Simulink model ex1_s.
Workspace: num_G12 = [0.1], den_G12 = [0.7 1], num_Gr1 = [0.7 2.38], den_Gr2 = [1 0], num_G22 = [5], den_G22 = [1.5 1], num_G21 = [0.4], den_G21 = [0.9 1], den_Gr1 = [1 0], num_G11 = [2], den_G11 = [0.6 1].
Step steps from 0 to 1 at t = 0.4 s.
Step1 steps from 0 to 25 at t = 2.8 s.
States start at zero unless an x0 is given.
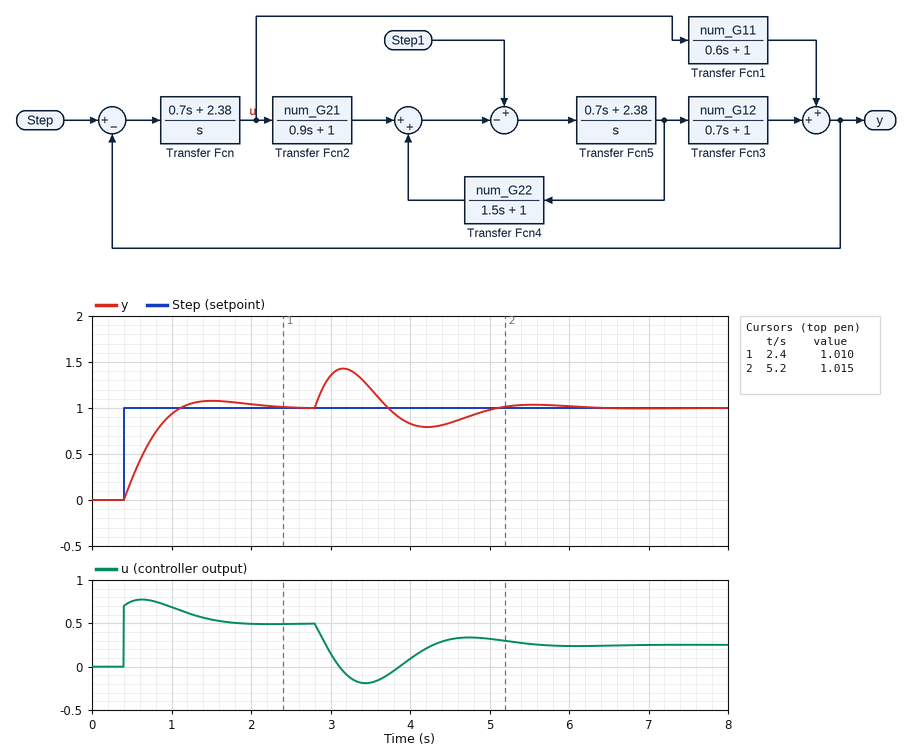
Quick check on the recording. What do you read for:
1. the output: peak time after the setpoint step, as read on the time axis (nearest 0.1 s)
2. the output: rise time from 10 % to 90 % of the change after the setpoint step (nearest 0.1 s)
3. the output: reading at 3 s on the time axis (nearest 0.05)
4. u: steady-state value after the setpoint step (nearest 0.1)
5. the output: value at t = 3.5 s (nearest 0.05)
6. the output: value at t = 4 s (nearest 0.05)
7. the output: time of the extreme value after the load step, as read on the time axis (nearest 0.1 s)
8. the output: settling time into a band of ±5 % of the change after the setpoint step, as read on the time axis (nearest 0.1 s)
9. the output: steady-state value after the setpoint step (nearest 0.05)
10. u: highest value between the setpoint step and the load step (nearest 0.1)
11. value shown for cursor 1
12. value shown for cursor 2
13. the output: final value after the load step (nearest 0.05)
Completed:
1.5 s
0.5 s
1.35
0.5
1.20
0.85
3.2 s
1.9 s
1.00
0.8
1.010
1.015
1.00
